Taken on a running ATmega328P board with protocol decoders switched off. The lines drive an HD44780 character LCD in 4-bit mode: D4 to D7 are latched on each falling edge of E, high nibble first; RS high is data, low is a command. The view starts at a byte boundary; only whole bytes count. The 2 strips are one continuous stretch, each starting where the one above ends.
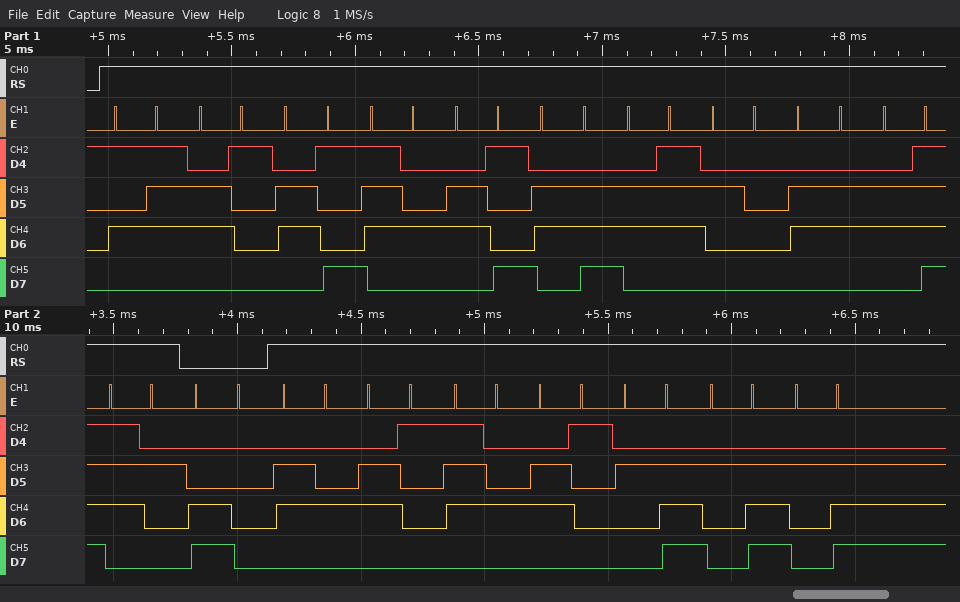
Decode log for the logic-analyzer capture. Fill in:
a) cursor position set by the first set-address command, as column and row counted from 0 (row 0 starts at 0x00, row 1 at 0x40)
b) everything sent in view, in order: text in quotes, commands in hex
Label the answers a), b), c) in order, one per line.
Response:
a) column 0, row 1
b) "Waiting for" 0xC0 "data..."
